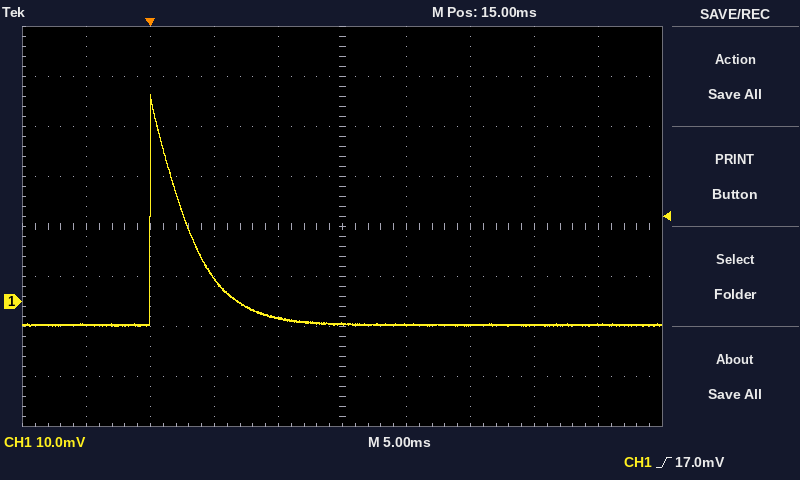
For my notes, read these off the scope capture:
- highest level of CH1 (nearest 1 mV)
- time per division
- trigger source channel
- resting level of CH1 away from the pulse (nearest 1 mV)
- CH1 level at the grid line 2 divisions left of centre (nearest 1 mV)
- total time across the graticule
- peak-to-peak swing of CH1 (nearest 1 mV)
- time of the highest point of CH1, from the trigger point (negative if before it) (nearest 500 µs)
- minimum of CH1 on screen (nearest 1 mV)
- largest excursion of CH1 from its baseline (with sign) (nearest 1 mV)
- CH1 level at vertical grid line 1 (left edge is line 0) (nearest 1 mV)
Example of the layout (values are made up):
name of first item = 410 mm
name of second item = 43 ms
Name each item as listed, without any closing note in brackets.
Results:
highest level of CH1 = 41 mV
time per division = 5 ms
trigger source channel = CH1
resting level of CH1 away from the pulse = -5 mV
CH1 level at the grid line 2 divisions left of centre = 5 mV
total time across the graticule = 50 ms
peak-to-peak swing of CH1 = 46 mV
time of the highest point of CH1, from the trigger point (negative if before it) = 0.0 ms
minimum of CH1 on screen = -5 mV
largest excursion of CH1 from its baseline (with sign) = +46 mV
CH1 level at vertical grid line 1 (left edge is line 0) = -5 mV
